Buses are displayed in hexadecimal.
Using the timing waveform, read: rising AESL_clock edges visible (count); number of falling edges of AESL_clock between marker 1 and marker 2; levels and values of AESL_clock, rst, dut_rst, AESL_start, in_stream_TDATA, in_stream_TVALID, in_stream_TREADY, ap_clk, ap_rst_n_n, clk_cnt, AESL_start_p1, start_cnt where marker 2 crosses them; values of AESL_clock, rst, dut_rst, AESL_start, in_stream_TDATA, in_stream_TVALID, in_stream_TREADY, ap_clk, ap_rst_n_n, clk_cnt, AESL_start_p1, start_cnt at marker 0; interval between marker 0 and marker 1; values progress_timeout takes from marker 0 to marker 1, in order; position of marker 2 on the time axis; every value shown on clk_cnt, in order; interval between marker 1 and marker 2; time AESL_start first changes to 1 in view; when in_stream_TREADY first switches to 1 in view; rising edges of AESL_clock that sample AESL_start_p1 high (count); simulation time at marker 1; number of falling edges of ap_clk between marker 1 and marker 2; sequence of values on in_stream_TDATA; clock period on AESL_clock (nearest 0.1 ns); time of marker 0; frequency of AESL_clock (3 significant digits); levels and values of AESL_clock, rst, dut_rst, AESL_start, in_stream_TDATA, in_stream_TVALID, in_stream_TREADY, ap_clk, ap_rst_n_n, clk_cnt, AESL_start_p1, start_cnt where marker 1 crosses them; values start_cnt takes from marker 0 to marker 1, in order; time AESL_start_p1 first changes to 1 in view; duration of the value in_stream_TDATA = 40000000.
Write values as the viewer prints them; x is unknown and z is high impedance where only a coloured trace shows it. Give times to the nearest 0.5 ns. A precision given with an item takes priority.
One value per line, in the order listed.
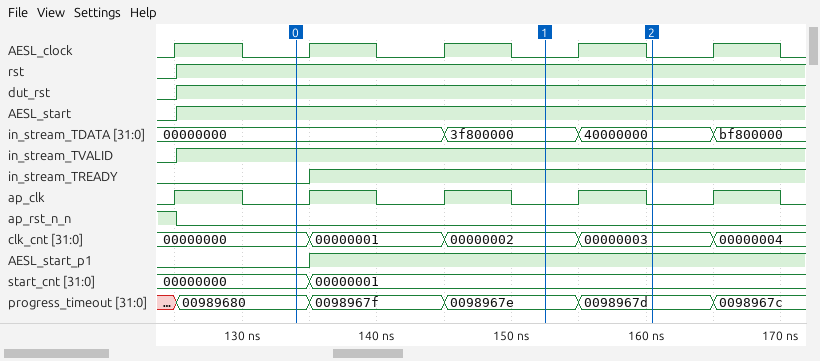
5
1
AESL_clock=0, rst=1, dut_rst=1, AESL_start=1, in_stream_TDATA=40000000, in_stream_TVALID=1, in_stream_TREADY=1, ap_clk=0, ap_rst_n_n=0, clk_cnt=00000003, AESL_start_p1=1, start_cnt=00000001
AESL_clock=0, rst=1, dut_rst=1, AESL_start=1, in_stream_TDATA=00000000, in_stream_TVALID=1, in_stream_TREADY=0, ap_clk=0, ap_rst_n_n=0, clk_cnt=00000000, AESL_start_p1=0, start_cnt=00000000
18.5 ns
00989680, 0098967f, 0098967e
160.5 ns
00000000, 00000001, 00000002, 00000003, 00000004
8 ns
125 ns
135 ns
3
152.5 ns
1
00000000, 3f800000, 40000000, bf800000
10 ns
134 ns
100 MHz
AESL_clock=0, rst=1, dut_rst=1, AESL_start=1, in_stream_TDATA=3f800000, in_stream_TVALID=1, in_stream_TREADY=1, ap_clk=0, ap_rst_n_n=0, clk_cnt=00000002, AESL_start_p1=1, start_cnt=00000001
00000000, 00000001
135 ns
10 ns
